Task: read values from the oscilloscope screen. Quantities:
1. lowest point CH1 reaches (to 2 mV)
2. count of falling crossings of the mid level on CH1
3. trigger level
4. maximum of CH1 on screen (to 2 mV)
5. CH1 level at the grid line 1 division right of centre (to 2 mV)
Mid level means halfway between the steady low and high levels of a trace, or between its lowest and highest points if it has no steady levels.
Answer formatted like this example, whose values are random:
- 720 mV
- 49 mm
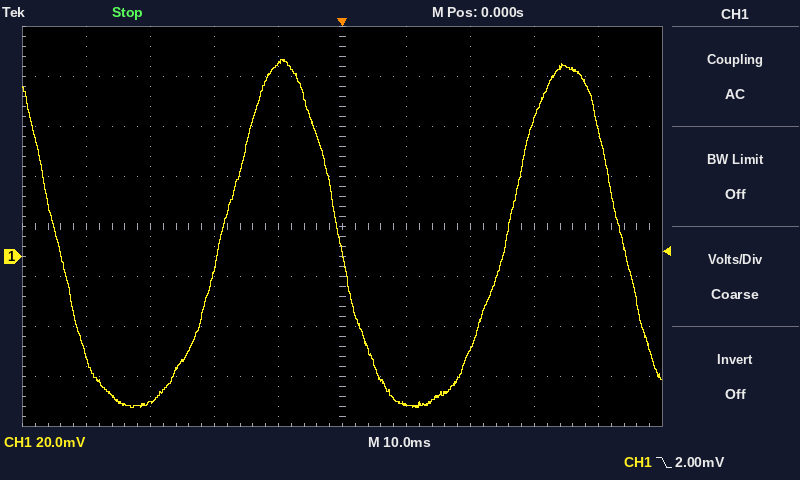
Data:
- -60 mV
- 3
- 2.00 mV
- 78 mV
- -60 mV
